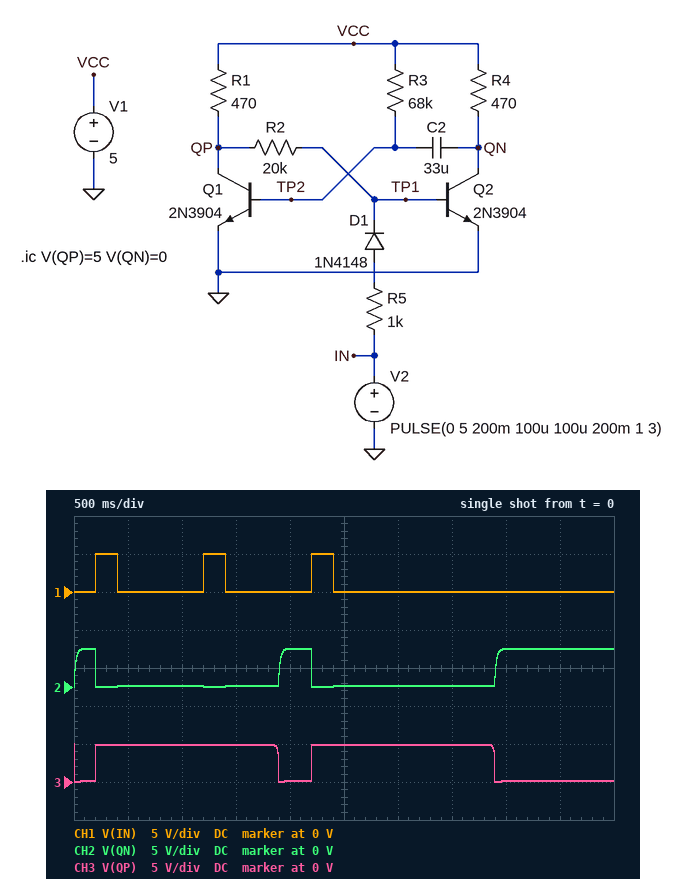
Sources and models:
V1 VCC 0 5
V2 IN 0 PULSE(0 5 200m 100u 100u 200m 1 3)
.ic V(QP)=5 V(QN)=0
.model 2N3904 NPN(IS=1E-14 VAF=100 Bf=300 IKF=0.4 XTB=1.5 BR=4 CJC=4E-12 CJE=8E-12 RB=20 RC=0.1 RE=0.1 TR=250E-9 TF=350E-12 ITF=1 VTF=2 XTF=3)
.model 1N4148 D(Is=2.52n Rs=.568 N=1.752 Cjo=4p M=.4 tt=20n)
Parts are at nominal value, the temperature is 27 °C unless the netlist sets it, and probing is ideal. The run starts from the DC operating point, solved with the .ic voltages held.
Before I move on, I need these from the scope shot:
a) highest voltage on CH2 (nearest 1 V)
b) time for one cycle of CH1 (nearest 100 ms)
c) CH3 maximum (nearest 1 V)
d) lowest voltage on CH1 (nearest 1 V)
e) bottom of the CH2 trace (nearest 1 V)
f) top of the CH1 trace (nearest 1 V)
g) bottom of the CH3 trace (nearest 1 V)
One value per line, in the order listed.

5 V
1.0 s
5 V
0 V
0 V
5 V
0 V
